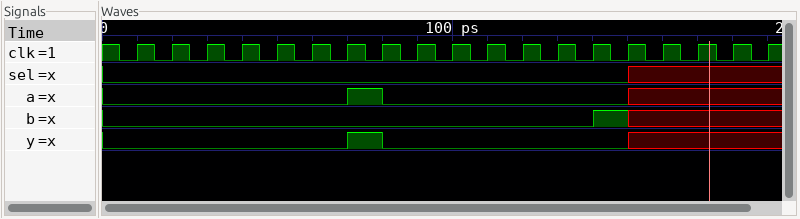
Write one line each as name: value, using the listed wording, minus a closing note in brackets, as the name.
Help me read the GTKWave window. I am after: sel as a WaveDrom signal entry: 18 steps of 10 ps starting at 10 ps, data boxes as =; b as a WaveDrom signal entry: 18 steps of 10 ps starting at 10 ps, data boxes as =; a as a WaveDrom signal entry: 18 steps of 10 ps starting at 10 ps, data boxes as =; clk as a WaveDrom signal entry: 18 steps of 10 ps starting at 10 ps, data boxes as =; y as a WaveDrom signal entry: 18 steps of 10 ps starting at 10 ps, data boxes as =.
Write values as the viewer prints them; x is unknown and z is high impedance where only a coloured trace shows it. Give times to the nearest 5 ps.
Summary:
sel as a WaveDrom signal entry: 18 steps of 10 ps starting at 10 ps, data boxes as =: {name: 'sel', wave: '0.............x...'}
b as a WaveDrom signal entry: 18 steps of 10 ps starting at 10 ps, data boxes as =: {name: 'b', wave: '0............1x...'}
a as a WaveDrom signal entry: 18 steps of 10 ps starting at 10 ps, data boxes as =: {name: 'a', wave: '0.....10......x...'}
clk as a WaveDrom signal entry: 18 steps of 10 ps starting at 10 ps, data boxes as =: {name: 'clk', wave: 'p.................'}
y as a WaveDrom signal entry: 18 steps of 10 ps starting at 10 ps, data boxes as =: {name: 'y', wave: '0.....10......x...'}
